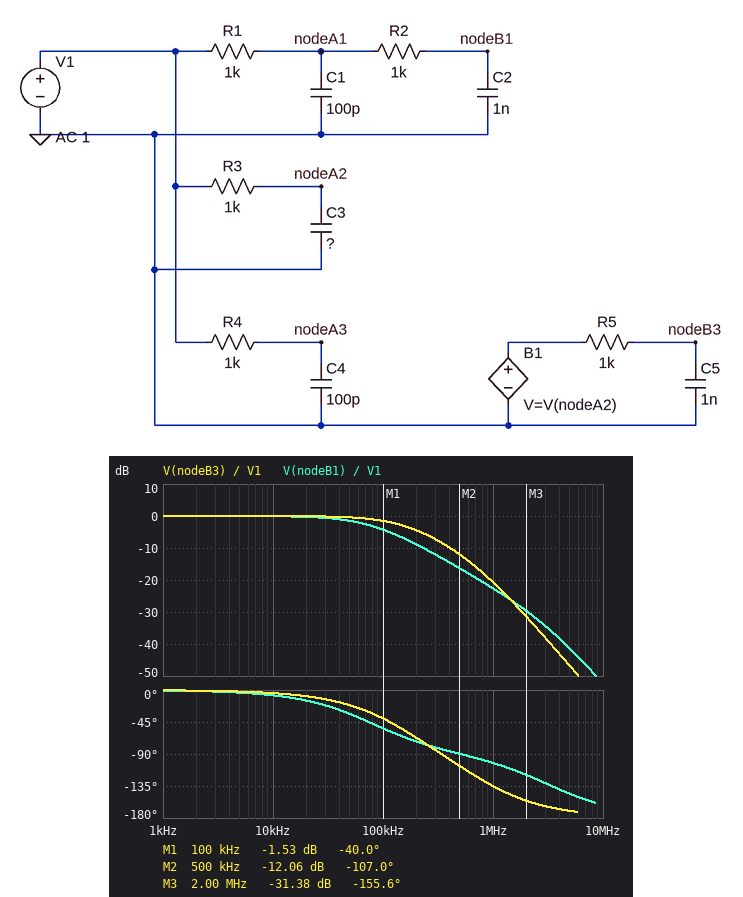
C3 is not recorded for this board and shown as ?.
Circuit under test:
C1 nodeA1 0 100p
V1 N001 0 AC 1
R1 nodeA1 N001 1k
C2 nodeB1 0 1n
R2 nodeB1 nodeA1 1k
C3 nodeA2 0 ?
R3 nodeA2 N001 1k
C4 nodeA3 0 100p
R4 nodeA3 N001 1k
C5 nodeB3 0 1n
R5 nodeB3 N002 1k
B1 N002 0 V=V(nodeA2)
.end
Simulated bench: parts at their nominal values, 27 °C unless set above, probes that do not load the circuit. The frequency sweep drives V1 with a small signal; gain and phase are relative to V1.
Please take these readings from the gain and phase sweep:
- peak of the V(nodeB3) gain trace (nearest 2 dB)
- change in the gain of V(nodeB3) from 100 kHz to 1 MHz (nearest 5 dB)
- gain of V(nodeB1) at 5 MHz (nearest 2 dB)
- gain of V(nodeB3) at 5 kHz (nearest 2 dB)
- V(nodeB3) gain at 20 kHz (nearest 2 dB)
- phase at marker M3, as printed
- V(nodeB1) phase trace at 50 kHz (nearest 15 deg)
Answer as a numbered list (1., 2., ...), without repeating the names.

1. 0 dB
2. -20 dB
3. -42 dB
4. 0 dB
5. 0 dB
6. -155.6 deg
7. -30 deg
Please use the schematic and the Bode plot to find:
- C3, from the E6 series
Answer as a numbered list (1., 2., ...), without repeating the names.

1. 220 pF
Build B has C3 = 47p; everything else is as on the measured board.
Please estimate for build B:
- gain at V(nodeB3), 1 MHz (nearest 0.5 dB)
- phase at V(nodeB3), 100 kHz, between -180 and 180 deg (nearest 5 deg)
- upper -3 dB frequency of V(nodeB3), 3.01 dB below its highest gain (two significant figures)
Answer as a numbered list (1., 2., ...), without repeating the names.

1. -16.5 dB
2. -35 deg
3. 160 kHz
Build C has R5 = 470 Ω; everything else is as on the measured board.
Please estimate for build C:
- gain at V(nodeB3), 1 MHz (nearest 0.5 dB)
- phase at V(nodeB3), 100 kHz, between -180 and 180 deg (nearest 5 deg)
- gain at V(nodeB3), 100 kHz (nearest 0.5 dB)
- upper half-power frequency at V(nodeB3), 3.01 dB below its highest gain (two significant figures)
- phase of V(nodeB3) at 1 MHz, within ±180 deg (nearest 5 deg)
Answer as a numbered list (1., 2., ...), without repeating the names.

1. -14.5 dB
2. -25 deg
3. -0.5 dB
4. 290 kHz
5. -125 deg
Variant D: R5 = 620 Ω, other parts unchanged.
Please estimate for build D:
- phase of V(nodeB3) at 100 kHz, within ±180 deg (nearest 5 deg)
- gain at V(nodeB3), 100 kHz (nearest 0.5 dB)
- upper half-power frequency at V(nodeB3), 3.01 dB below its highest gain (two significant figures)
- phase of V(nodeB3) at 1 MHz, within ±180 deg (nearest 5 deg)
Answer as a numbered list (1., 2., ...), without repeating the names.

1. -30 deg
2. -0.5 dB
3. 230 kHz
4. -130 deg
